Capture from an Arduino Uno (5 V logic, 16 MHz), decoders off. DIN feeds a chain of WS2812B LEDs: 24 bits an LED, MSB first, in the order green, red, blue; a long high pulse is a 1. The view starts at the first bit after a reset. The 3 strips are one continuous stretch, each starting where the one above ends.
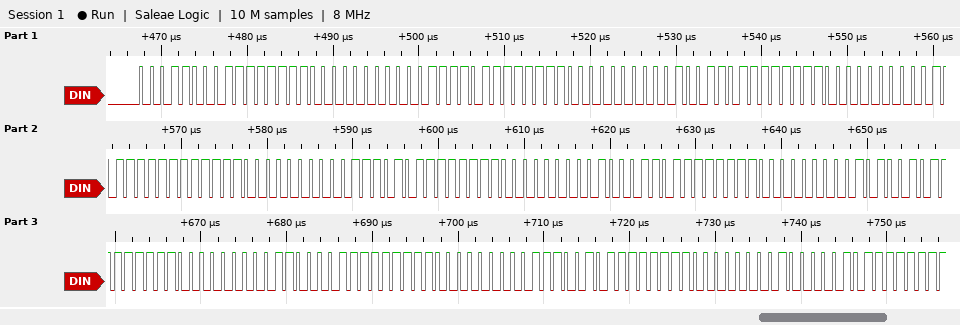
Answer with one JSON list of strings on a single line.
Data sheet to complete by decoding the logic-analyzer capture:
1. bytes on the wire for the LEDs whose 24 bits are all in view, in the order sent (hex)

["18 FF 00 1E FF 00 26 FF 00 2F FF 00 3A FF 00 46 FF 00 52 FF 00 61 FF 00 72 FF 00"]
